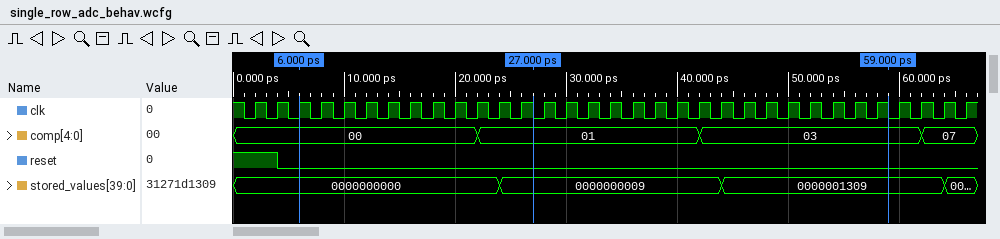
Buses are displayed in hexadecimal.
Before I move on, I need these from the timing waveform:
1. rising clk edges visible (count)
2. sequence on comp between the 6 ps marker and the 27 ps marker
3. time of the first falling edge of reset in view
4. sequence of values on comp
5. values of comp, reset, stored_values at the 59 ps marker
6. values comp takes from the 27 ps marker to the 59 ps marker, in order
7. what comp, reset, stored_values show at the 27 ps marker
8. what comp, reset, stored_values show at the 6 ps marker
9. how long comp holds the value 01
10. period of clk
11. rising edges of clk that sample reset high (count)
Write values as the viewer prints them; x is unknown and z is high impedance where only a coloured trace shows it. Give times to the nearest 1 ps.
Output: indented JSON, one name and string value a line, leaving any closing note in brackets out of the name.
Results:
{
  "rising clk edges visible": "33",
  "sequence on comp between the 6 ps marker and the 27 ps marker": "00, 01",
  "time of the first falling edge of reset in view": "4 ps",
  "sequence of values on comp": "00, 01, 03, 07",
  "values of comp, reset, stored_values at the 59 ps marker": "comp=03, reset=0, stored_values=0000001309",
  "values comp takes from the 27 ps marker to the 59 ps marker, in order": "01, 03",
  "what comp, reset, stored_values show at the 27 ps marker": "comp=01, reset=0, stored_values=0000000009",
  "what comp, reset, stored_values show at the 6 ps marker": "comp=00, reset=0, stored_values=0000000000",
  "how long comp holds the value 01": "20 ps",
  "period of clk": "2 ps",
  "rising edges of clk that sample reset high": "2"
}
